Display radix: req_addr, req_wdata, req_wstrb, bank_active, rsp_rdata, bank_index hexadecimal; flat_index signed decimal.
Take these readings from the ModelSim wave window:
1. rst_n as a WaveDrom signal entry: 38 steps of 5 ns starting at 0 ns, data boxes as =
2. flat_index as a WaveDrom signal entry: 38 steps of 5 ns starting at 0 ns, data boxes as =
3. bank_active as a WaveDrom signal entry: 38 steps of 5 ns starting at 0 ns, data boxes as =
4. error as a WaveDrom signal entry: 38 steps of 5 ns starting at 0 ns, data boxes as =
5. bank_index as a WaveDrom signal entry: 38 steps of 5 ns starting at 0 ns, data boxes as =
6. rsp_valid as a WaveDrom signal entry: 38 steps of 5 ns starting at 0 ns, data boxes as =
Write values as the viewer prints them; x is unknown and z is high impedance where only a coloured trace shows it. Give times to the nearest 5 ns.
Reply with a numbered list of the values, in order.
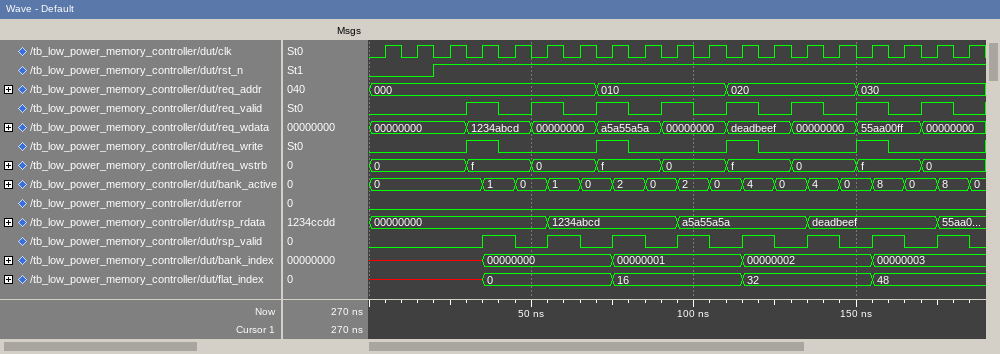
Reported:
1. {name: 'rst_n', wave: '0...1.................................'}
2. {name: 'flat_index', wave: 'x......=.......=.......=.......=......', data: '0 16 32 48'}
3. {name: 'bank_active', wave: '=......=.=.=.=.=.=.=.=.=.=.=.=.=.=.=.=', data: '0 1 0 1 0 2 0 2 0 4 0 4 0 8 0 8 0'}
4. {name: 'error', wave: '0.....................................'}
5. {name: 'bank_index', wave: 'x......=.......=.......=.......=......', data: '00000000 00000001 00000002 00000003'}
6. {name: 'rsp_valid', wave: '0......1.0.1.0.1.0.1.0.1.0.1.0.1.0.1.0'}
